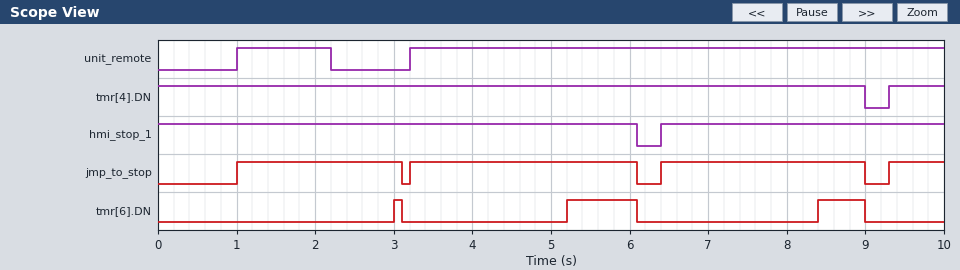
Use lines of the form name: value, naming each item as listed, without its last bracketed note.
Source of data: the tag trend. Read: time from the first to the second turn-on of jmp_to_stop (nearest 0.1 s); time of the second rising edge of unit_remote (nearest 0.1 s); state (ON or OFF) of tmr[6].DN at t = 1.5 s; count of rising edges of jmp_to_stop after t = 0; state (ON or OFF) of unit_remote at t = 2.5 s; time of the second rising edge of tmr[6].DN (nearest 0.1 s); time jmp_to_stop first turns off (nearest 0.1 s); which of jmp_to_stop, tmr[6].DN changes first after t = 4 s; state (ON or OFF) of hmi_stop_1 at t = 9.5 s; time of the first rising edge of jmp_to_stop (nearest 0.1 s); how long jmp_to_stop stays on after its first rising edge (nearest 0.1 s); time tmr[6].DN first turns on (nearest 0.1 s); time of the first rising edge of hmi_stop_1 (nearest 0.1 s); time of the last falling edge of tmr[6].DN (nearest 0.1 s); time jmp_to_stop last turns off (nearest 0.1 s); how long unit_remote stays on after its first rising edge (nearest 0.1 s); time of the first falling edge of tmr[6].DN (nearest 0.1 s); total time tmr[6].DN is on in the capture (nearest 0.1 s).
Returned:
time from the first to the second turn-on of jmp_to_stop: 2.2 s
time of the second rising edge of unit_remote: 3.2 s
state (ON or OFF) of tmr[6].DN at t = 1.5 s: OFF
count of rising edges of jmp_to_stop after t = 0: 4
state (ON or OFF) of unit_remote at t = 2.5 s: OFF
time of the second rising edge of tmr[6].DN: 5.2 s
time jmp_to_stop first turns off: 3.1 s
which of jmp_to_stop, tmr[6].DN changes first after t = 4 s: tmr[6].DN
state (ON or OFF) of hmi_stop_1 at t = 9.5 s: ON
time of the first rising edge of jmp_to_stop: 1.0 s
how long jmp_to_stop stays on after its first rising edge: 2.1 s
time tmr[6].DN first turns on: 3.0 s
time of the first rising edge of hmi_stop_1: 6.4 s
time of the last falling edge of tmr[6].DN: 9.0 s
time jmp_to_stop last turns off: 9.0 s
how long unit_remote stays on after its first rising edge: 1.2 s
time of the first falling edge of tmr[6].DN: 3.1 s
total time tmr[6].DN is on in the capture: 1.6 s
